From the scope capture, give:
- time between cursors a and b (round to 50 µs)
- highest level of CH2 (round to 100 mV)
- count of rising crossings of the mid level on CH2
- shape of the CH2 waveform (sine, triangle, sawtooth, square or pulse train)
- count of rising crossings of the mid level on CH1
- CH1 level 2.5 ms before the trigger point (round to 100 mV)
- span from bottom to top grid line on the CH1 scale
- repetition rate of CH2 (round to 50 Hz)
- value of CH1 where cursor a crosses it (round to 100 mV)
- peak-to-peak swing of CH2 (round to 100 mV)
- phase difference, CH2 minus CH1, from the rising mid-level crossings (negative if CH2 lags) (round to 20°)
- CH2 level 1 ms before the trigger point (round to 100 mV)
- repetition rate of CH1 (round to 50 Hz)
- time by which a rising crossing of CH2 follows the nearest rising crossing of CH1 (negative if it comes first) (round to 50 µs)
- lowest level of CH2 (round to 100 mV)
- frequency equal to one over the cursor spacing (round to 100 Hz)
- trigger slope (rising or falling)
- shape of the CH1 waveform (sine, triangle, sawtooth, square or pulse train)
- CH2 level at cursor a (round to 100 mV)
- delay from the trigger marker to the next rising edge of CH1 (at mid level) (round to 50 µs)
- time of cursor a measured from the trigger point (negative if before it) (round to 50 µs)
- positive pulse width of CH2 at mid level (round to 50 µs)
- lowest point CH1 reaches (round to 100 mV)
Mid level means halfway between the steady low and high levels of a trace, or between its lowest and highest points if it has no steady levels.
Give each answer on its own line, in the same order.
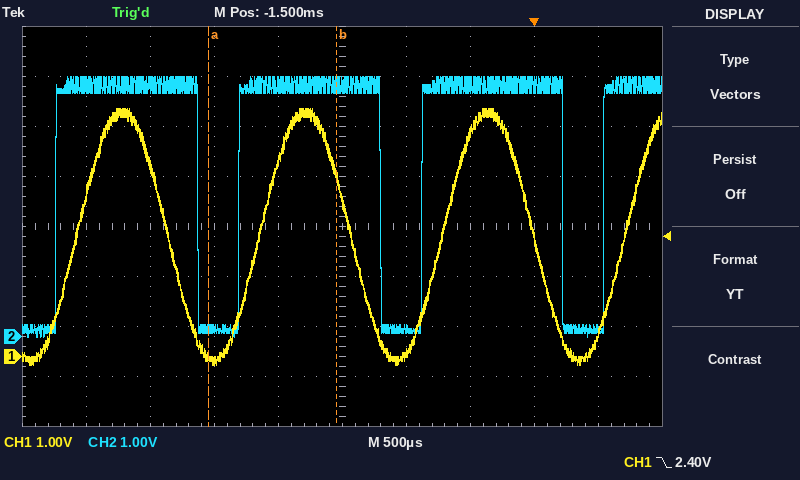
1.00 ms
5.2 V
4
pulse train
4
-100 mV
8 V
700 Hz
0.0 V
5.2 V
+40°
200 mV
700 Hz
-150 µs
0.0 V
1.0 kHz
falling
sine
200 mV
700 µs
-2.55 ms
1.10 ms
-200 mV
